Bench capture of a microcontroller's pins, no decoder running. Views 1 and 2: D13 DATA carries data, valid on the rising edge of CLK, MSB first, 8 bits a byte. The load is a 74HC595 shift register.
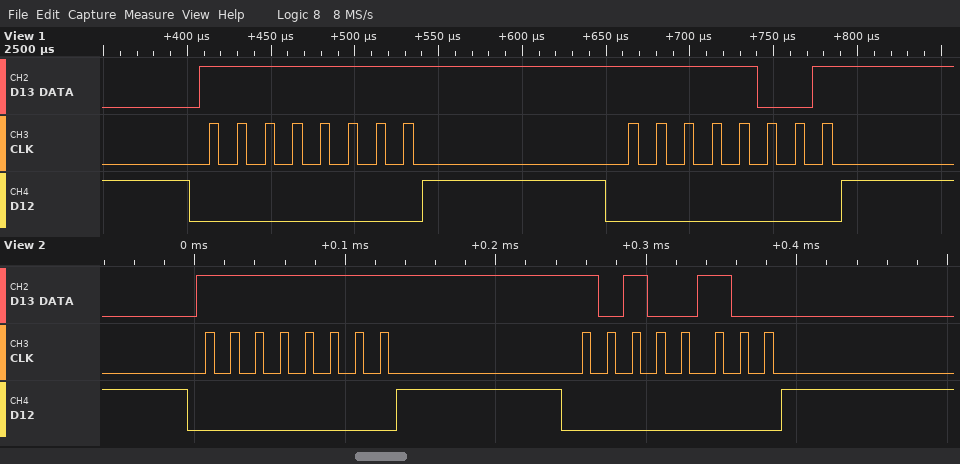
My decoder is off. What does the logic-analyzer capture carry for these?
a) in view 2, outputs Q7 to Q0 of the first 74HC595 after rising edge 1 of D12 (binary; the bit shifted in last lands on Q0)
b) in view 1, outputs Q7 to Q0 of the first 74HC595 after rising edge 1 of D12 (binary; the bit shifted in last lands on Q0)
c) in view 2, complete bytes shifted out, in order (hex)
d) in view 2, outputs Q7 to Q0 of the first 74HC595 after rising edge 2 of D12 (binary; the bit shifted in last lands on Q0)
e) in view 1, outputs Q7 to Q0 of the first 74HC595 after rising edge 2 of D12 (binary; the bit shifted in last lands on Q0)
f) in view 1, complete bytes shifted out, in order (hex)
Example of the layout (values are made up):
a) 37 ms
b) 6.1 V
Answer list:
a) 11111111
b) 11111111
c) FF A4
d) 10100100
e) 11111001
f) FF F9
